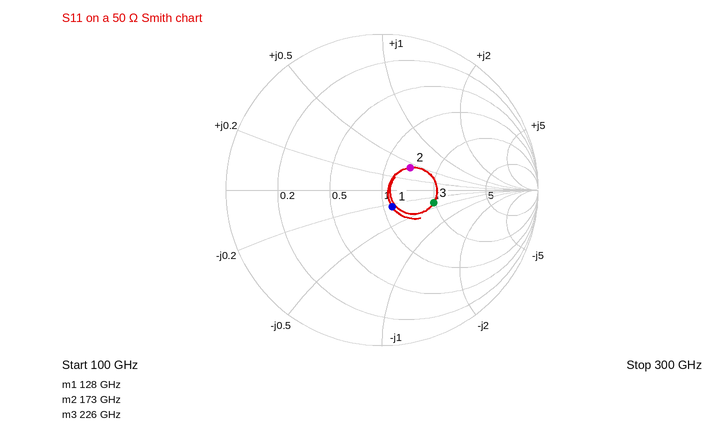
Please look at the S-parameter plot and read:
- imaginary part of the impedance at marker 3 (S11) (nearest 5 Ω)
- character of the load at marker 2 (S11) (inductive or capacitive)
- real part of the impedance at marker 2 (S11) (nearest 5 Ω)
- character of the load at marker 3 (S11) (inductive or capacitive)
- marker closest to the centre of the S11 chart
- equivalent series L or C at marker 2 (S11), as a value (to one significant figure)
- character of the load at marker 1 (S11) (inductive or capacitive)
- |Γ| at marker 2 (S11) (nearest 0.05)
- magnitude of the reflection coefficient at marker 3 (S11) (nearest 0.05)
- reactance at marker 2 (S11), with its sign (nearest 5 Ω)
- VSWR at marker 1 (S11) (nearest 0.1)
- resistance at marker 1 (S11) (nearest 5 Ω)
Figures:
-20 Ω
inductive
70 Ω
capacitive
marker 1
20 pH
capacitive
0.25
0.35
+20 Ω
1.3
55 Ω
